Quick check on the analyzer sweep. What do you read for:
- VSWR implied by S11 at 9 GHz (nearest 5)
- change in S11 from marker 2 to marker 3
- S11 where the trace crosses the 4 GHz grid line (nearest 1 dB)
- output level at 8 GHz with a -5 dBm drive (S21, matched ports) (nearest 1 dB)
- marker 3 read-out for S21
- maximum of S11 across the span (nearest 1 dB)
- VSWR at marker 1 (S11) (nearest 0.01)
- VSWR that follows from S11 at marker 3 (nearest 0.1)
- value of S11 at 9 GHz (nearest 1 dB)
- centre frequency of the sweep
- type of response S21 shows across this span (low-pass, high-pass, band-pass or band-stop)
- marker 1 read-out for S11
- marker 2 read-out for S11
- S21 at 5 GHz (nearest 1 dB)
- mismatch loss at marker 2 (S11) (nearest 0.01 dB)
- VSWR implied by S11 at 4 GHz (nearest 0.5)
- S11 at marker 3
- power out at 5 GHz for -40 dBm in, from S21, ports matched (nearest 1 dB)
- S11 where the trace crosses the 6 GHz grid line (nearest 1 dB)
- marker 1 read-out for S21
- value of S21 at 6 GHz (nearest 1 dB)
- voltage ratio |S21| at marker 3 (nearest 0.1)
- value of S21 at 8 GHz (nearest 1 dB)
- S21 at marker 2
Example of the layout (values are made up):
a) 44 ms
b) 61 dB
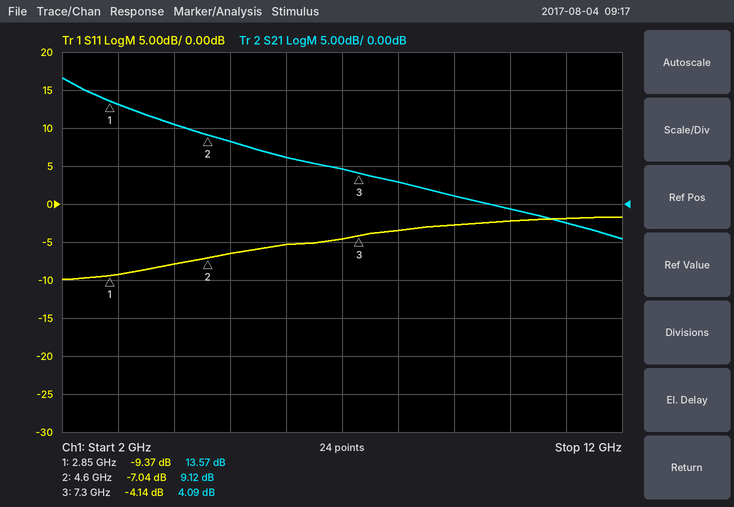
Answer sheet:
a) 5
b) 2.90 dB
c) -8 dB
d) -2 dBm
e) 4.09 dB
f) -2 dB
g) 2.03
h) 4.3
i) -3 dB
j) 7 GHz
k) low-pass
l) -9.37 dB
m) -7.04 dB
n) 8 dB
o) 0.96 dB
p) 2.5
q) -4.14 dB
r) -32 dBm
s) -5 dB
t) 13.57 dB
u) 6 dB
v) 1.6
w) 3 dB
x) 9.12 dB
